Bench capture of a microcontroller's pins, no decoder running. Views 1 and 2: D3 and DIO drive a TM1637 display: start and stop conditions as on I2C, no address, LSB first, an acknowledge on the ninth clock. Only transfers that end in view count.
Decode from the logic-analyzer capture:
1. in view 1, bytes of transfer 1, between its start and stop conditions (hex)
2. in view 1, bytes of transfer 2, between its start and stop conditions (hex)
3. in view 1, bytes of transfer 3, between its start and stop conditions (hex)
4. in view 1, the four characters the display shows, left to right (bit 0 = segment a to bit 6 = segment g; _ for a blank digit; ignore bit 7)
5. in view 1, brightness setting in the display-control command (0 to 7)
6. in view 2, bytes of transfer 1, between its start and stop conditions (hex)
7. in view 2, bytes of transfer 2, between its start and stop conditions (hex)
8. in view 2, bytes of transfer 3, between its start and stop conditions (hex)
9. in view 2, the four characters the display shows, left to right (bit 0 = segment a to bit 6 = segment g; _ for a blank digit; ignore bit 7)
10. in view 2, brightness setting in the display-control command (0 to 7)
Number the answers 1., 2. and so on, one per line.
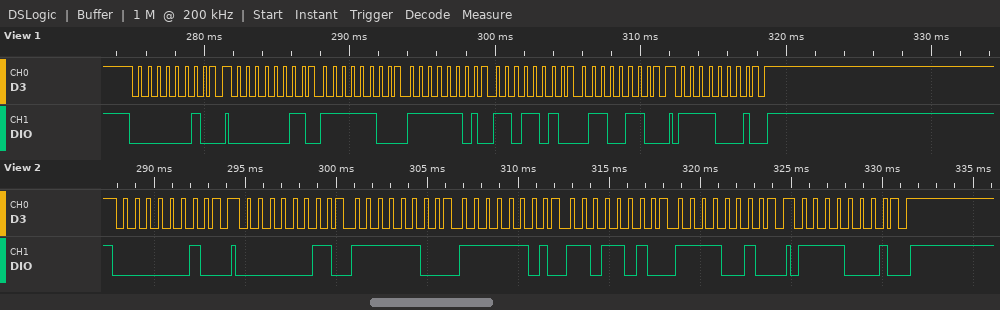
1. 40
2. C0 3F BF 5B 66
3. 8F
4. 0024
5. 7
6. 40
7. C0 3F BF 5B 4F
8. 8F
9. 0023
10. 7
